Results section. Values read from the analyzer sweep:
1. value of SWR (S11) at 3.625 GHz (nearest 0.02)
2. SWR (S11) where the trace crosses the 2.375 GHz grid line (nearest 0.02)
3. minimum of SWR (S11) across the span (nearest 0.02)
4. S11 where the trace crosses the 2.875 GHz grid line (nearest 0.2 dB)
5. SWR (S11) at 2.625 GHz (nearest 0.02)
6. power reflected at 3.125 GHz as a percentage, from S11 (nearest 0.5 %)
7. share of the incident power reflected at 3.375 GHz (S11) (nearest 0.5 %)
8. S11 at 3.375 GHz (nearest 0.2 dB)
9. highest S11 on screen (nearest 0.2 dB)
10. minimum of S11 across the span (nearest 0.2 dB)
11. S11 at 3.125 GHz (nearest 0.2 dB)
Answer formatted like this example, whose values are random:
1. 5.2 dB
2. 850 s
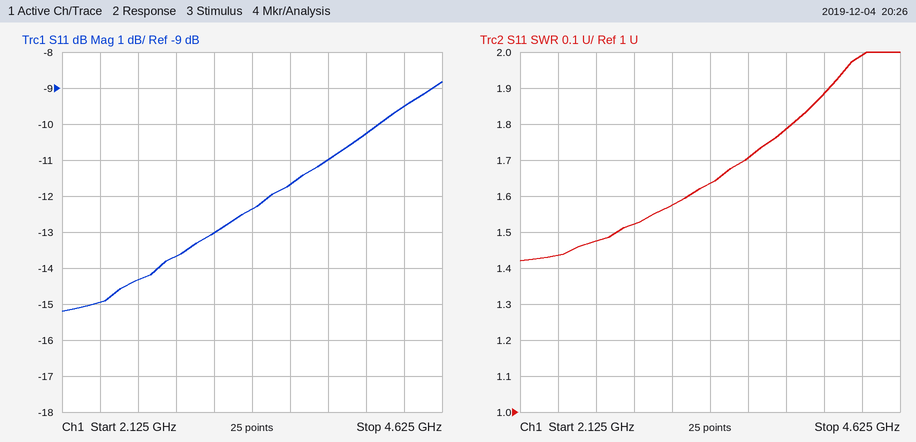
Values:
1. 1.70
2. 1.44
3. 1.42
4. -13.6 dB
5. 1.48
6. 5.0 %
7. 6.0 %
8. -12.4 dB
9. -8.8 dB
10. -15.2 dB
11. -13.0 dB
